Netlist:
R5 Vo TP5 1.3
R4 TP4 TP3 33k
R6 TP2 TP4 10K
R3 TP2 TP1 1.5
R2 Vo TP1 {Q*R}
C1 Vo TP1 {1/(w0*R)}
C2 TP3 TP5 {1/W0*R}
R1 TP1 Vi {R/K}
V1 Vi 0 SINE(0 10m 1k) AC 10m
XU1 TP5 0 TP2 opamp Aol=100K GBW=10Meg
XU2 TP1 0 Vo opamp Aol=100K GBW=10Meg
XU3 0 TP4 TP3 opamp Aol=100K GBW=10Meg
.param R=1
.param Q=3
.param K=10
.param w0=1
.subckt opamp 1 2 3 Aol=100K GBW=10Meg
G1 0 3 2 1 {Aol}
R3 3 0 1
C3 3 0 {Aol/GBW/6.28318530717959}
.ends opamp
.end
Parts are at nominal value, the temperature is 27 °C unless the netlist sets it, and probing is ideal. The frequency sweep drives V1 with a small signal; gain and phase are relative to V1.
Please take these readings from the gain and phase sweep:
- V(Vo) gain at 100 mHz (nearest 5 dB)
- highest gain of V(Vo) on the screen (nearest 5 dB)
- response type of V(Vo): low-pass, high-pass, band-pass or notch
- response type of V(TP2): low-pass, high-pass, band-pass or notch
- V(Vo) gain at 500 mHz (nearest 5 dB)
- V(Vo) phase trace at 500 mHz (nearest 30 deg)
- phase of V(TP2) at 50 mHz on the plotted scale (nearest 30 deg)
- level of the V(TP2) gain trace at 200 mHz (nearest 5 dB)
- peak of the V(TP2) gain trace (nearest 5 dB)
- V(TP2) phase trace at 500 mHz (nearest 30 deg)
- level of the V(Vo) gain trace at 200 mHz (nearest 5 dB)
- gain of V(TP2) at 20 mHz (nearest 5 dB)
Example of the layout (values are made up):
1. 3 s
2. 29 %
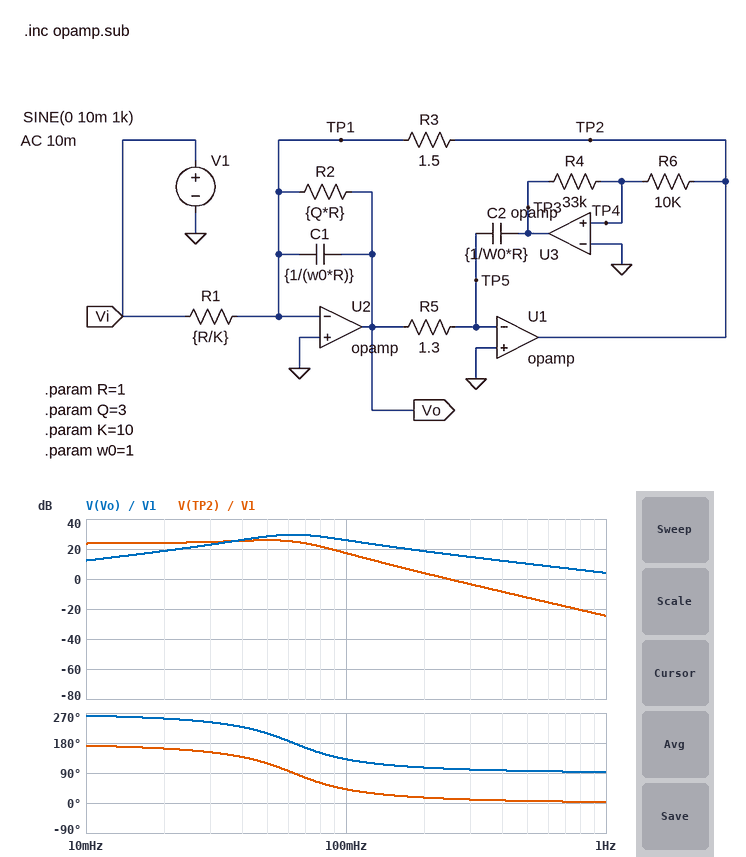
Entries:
1. 25 dB
2. 30 dB
3. band-pass
4. low-pass
5. 10 dB
6. 90 deg
7. 120 deg
8. 5 dB
9. 25 dB
10. 0 deg
11. 20 dB
12. 25 dB
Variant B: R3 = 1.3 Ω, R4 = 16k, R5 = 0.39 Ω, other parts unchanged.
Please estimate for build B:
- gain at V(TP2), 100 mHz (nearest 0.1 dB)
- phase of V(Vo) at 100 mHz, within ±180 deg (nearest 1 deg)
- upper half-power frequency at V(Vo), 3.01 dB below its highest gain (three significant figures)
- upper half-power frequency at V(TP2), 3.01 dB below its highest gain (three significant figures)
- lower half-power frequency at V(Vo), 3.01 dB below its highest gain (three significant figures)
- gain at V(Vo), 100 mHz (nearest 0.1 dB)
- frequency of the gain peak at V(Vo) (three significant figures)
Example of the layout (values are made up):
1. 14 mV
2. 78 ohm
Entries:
1. 25.4 dB
2. -104 deg
3. 205 mHz
4. 198 mHz
5. 152 mHz
6. 17.2 dB
7. 177 mHz
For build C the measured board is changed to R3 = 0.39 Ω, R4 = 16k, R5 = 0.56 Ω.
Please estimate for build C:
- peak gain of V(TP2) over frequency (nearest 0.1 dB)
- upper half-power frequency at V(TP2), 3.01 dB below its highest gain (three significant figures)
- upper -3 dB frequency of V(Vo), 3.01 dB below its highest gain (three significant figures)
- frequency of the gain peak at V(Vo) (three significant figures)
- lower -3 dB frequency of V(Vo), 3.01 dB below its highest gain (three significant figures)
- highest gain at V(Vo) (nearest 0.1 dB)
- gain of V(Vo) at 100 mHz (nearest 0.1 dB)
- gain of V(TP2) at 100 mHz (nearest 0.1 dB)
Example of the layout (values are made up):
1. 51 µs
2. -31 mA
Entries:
1. 26.0 dB
2. 292 mHz
3. 297 mHz
4. 269 mHz
5. 244 mHz
6. 29.5 dB
7. 8.1 dB
8. 13.1 dB
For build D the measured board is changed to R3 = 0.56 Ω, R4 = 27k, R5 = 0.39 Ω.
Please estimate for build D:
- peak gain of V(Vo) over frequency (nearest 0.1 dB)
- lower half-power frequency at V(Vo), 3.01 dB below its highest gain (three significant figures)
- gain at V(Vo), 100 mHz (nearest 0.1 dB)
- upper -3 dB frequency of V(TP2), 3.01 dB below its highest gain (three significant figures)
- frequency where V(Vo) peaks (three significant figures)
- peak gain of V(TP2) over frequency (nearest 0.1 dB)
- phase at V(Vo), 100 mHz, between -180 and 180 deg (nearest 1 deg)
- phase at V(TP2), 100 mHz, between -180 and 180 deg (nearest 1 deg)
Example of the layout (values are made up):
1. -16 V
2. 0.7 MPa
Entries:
1. 29.5 dB
2. 182 mHz
3. 13.6 dB
4. 229 mHz
5. 207 mHz
6. 26.9 dB
7. -99 deg
8. 171 deg
